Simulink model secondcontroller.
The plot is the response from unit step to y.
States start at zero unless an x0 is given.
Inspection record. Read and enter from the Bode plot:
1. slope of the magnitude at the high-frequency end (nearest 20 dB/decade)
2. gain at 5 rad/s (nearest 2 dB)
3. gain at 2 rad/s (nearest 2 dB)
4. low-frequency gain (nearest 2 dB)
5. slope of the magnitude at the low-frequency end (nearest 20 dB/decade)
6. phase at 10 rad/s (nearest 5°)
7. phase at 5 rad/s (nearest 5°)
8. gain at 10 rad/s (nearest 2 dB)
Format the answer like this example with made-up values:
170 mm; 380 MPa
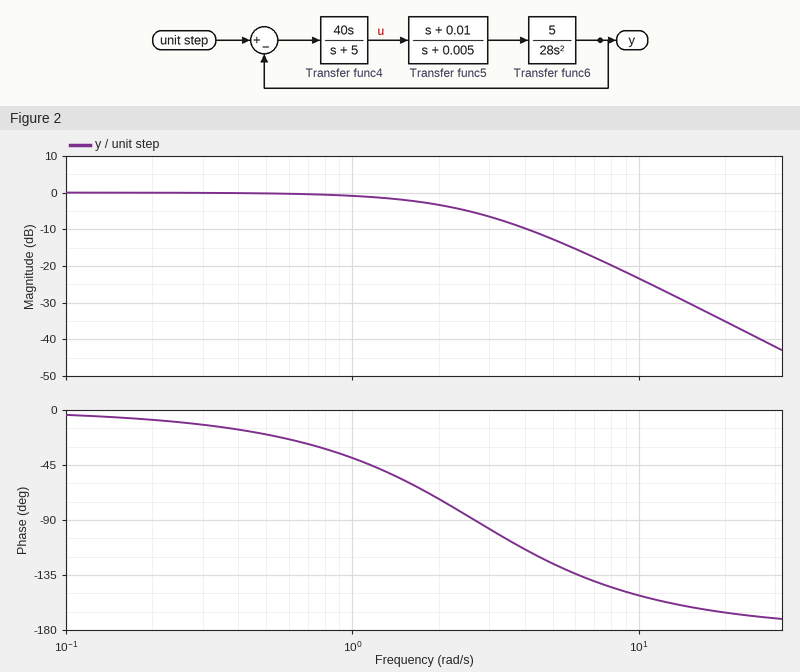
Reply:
-40 dB/decade; -12 dB; -4 dB; 0 dB; 0 dB/decade; -150°; -125°; -24 dB
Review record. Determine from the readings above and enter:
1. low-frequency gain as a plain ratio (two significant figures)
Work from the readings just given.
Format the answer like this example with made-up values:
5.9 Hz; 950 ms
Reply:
1.0
